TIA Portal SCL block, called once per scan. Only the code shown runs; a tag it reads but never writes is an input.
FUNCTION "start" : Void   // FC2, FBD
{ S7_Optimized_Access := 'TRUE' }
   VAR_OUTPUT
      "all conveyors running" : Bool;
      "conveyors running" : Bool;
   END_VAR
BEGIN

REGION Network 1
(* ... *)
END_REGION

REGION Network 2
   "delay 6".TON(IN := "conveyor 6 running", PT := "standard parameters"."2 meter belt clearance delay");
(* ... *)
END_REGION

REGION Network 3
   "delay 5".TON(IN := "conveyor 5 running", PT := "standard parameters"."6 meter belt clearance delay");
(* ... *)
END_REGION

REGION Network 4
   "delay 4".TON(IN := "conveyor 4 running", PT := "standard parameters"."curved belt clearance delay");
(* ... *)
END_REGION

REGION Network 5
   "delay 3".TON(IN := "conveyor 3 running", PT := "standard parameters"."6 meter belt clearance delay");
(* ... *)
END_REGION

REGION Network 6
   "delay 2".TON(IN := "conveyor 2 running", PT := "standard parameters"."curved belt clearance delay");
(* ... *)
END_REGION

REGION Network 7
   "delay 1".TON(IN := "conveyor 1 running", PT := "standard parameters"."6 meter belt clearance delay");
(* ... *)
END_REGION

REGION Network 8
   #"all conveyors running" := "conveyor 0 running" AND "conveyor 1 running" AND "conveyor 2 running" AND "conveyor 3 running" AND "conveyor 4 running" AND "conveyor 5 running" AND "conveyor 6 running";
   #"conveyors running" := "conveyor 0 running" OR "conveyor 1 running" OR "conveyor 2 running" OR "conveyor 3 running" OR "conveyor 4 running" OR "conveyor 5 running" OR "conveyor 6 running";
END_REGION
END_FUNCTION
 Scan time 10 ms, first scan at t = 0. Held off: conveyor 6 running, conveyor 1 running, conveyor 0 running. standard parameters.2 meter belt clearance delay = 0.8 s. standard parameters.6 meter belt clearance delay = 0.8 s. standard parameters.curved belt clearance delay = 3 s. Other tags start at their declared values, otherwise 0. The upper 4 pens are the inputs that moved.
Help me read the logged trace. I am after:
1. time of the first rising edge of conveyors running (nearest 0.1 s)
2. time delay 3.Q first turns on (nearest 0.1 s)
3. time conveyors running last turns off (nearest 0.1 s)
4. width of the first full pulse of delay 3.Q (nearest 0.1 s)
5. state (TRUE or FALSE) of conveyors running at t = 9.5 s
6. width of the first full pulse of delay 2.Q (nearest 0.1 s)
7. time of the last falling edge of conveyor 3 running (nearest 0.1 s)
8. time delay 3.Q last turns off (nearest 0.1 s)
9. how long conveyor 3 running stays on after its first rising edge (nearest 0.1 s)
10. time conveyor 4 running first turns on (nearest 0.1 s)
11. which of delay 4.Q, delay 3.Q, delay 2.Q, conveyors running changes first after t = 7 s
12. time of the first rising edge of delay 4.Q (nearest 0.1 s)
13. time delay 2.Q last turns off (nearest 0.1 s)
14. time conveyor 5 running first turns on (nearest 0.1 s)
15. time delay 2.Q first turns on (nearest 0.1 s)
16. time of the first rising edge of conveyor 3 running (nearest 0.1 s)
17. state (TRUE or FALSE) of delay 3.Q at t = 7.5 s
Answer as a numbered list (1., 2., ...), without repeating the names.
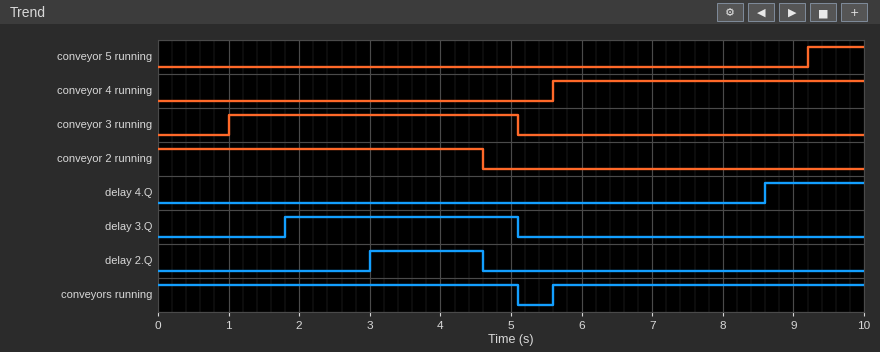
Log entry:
1. 5.6 s
2. 1.8 s
3. 5.1 s
4. 3.3 s
5. TRUE
6. 1.6 s
7. 5.1 s
8. 5.1 s
9. 4.1 s
10. 5.6 s
11. delay 4.Q
12. 8.6 s
13. 4.6 s
14. 9.2 s
15. 3.0 s
16. 1.0 s
17. FALSE
